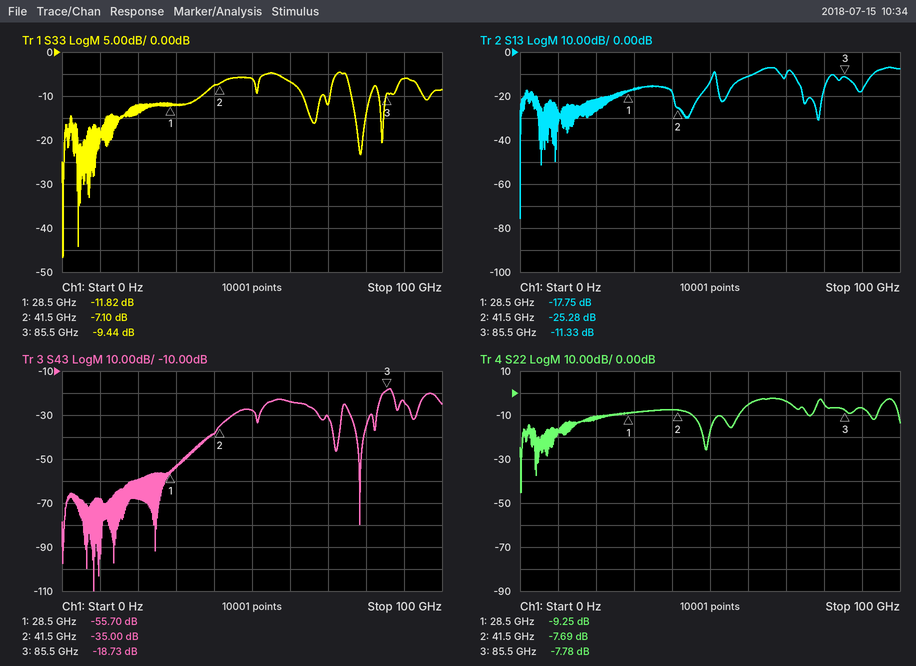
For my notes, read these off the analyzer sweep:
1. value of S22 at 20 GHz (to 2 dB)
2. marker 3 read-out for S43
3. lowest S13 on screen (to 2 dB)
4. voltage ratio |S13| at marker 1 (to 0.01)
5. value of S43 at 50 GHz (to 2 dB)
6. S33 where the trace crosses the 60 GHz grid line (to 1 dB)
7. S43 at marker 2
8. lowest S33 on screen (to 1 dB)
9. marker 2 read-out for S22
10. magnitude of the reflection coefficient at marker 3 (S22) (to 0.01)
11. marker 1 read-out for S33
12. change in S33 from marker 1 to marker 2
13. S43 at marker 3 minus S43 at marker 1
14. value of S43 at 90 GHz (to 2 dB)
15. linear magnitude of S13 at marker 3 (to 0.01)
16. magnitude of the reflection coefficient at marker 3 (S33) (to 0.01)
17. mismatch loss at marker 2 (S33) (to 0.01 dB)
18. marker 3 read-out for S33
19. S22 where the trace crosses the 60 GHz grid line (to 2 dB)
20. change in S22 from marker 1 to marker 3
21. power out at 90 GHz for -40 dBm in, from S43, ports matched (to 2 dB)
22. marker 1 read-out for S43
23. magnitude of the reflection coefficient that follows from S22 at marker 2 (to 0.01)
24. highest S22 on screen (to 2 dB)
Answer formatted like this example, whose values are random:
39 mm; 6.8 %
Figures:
-12 dB; -18.73 dB; -76 dB; 0.13; -28 dB; -7 dB; -35.00 dB; -47 dB; -7.69 dB; 0.41; -11.82 dB; 4.72 dB; 36.97 dB; -24 dB; 0.27; 0.34; 0.94 dB; -9.44 dB; -6 dB; 1.47 dB; -64 dBm; -55.70 dB; 0.41; -2 dB
